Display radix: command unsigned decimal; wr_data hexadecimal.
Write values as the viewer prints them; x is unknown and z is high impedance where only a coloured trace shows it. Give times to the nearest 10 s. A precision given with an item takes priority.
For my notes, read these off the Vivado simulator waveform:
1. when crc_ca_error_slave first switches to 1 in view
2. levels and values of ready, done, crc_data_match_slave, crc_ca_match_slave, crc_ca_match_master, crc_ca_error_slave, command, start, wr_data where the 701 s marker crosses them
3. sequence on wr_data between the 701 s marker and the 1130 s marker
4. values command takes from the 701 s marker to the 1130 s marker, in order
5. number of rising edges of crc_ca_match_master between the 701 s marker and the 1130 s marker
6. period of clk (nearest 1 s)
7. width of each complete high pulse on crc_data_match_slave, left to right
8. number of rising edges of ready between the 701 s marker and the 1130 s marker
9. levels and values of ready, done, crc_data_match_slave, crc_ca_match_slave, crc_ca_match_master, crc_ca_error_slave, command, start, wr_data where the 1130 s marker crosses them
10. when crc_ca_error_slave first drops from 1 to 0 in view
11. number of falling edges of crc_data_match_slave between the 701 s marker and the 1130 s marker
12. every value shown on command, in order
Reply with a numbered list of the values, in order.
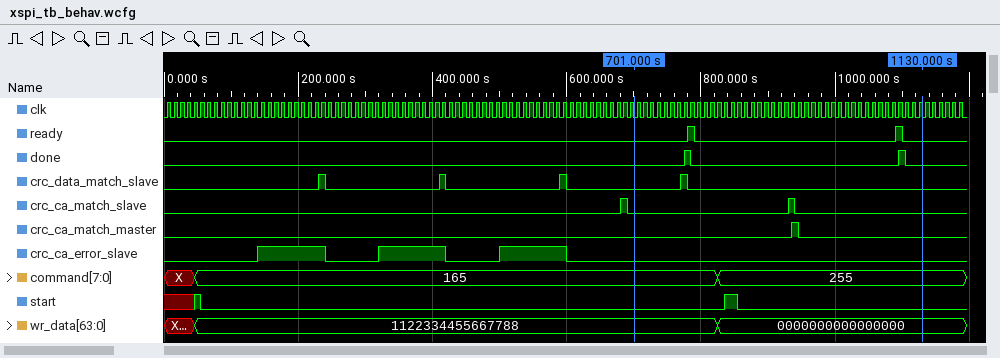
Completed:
1. 140 s
2. ready=0, done=0, crc_data_match_slave=0, crc_ca_match_slave=0, crc_ca_match_master=0, crc_ca_error_slave=0, command=165, start=0, wr_data=1122334455667788
3. 1122334455667788, 0000000000000000
4. 165, 255
5. 1
6. 10 s
7. 10 s, 10 s, 10 s, 10 s
8. 2
9. ready=0, done=0, crc_data_match_slave=0, crc_ca_match_slave=0, crc_ca_match_master=0, crc_ca_error_slave=0, command=255, start=0, wr_data=0000000000000000
10. 240 s
11. 1
12. X, 165, 255
